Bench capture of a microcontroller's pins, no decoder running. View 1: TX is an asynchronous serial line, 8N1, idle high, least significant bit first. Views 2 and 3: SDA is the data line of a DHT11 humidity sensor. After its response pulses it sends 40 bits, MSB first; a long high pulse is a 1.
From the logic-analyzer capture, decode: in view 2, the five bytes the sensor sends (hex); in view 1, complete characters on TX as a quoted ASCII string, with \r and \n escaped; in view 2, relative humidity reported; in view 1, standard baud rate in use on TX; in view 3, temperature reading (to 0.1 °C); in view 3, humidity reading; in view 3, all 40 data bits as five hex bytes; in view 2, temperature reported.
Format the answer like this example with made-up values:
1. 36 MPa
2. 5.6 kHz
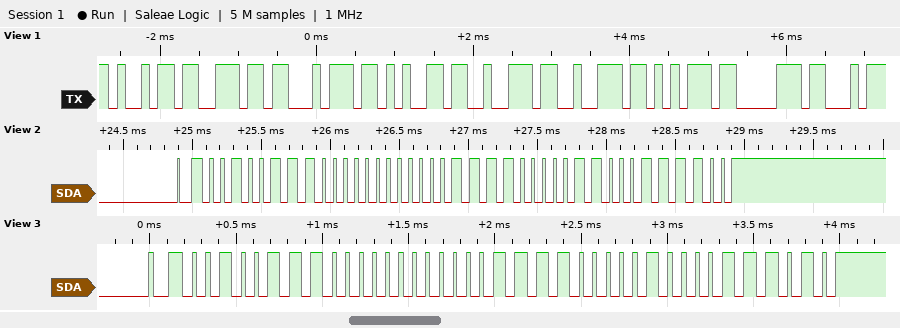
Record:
1. 27 00 0F 06 3C
2. "interrup"
3. 39 %
4. 9600 baud
5. 15.4 °C
6. 39 %
7. 27 00 0F 04 3A
8. 15.6 °C
